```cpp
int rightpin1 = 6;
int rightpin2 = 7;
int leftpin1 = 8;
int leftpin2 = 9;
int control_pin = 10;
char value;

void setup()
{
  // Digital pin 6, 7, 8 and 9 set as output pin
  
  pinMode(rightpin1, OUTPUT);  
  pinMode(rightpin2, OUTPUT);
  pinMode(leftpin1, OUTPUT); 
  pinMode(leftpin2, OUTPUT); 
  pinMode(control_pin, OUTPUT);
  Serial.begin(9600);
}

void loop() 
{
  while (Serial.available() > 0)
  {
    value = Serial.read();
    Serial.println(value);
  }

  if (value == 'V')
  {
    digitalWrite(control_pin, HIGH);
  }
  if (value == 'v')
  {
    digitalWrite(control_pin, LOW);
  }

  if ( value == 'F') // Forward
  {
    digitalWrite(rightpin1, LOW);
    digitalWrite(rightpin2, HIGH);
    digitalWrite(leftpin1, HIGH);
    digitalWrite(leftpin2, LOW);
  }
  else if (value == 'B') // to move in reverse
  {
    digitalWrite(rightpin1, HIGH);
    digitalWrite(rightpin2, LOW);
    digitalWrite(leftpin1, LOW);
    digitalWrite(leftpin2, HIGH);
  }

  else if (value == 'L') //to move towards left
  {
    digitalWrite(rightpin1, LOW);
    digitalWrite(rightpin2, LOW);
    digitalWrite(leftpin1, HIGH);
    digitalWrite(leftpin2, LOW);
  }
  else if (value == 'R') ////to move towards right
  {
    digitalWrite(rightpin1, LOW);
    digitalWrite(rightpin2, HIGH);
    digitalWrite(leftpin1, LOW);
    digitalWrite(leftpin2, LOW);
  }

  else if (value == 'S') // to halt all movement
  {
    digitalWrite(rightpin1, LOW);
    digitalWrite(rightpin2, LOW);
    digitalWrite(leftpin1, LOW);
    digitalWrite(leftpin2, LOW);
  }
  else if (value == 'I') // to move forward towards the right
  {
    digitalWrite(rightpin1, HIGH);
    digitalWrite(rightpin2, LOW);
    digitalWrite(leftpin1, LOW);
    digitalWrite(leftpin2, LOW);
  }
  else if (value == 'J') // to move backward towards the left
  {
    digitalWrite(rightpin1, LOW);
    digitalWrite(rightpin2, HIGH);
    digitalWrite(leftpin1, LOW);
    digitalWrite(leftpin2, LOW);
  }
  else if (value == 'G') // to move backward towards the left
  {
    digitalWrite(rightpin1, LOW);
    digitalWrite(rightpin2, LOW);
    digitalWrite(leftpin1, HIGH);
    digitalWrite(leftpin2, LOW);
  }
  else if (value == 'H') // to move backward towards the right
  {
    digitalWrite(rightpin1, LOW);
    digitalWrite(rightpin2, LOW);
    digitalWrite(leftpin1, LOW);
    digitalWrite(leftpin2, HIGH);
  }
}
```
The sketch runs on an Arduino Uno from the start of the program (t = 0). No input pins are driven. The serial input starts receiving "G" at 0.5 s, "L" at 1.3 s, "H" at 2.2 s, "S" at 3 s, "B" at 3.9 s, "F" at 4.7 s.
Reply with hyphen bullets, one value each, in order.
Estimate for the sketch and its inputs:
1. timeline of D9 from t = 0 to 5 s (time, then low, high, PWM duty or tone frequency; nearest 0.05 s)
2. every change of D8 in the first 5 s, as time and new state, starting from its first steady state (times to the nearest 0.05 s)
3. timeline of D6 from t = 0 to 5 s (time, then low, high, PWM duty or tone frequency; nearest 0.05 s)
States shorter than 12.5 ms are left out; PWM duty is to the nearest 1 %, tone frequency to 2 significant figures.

- 0 s low; 2.2 s high; 3 s low; 3.9 s high; 4.7 s low
- 0 s low; 0.5 s high; 2.2 s low; 4.7 s high
- 0 s low; 3.9 s high; 4.7 s low
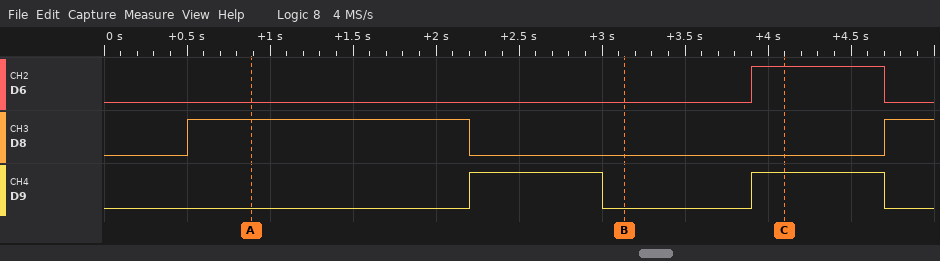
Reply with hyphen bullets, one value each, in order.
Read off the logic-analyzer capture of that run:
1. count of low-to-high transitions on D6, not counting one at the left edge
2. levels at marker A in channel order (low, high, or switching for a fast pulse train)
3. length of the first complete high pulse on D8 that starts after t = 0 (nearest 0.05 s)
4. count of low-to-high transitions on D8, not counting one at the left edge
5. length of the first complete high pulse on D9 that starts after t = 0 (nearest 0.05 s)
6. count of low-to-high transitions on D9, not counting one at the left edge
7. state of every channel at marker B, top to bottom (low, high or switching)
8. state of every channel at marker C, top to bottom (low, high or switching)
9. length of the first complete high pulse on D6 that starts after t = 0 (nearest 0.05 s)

- 1
- D6 low, D8 high, D9 low
- 1.70 s
- 2
- 0.80 s
- 2
- D6 low, D8 low, D9 low
- D6 high, D8 low, D9 high
- 0.80 s
